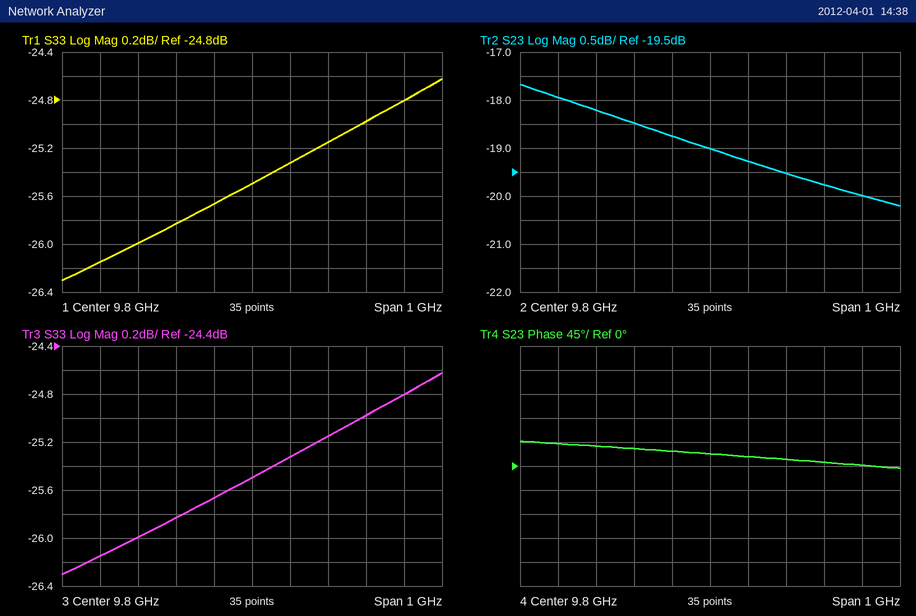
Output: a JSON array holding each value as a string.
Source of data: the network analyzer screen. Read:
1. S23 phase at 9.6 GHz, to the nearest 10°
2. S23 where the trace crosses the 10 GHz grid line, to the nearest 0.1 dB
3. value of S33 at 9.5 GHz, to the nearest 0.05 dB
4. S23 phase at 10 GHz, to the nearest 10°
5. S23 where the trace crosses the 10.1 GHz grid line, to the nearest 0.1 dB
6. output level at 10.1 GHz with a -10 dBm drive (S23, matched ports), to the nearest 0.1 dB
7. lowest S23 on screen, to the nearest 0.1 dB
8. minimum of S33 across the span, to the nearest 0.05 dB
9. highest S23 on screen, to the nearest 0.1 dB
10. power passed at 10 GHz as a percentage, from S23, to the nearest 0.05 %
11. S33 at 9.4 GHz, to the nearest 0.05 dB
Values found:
["30°", "-19.5 dB", "-26.00 dB", "10°", "-19.8 dB", "-29.8 dBm", "-20.2 dB", "-26.30 dB", "-17.7 dB", "1.10 %", "-26.15 dB"]
